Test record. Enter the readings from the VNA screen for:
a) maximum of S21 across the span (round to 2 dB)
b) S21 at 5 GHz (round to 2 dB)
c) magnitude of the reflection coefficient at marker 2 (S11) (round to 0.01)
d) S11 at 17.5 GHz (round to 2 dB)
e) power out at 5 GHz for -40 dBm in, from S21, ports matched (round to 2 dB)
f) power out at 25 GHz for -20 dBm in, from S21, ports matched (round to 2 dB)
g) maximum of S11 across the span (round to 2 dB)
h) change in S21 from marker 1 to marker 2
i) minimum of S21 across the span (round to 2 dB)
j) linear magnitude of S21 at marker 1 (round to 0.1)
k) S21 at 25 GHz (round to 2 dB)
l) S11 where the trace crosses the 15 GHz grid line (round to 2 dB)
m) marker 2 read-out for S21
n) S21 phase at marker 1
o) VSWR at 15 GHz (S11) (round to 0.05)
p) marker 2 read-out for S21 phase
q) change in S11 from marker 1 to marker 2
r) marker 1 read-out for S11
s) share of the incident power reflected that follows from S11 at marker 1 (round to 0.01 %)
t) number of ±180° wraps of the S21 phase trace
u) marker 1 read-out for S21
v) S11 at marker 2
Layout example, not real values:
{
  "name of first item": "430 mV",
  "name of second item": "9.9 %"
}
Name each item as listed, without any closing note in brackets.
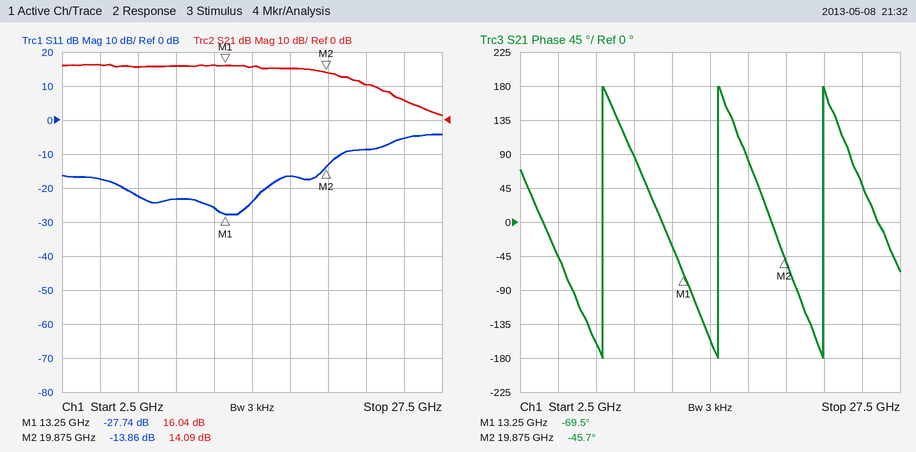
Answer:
{
  "maximum of S21 across the span": "16 dB",
  "S21 at 5 GHz": "16 dB",
  "magnitude of the reflection coefficient at marker 2 (S11)": "0.20",
  "S11 at 17.5 GHz": "-16 dB",
  "power out at 5 GHz for -40 dBm in, from S21, ports matched": "-24 dBm",
  "power out at 25 GHz for -20 dBm in, from S21, ports matched": "-14 dBm",
  "maximum of S11 across the span": "-4 dB",
  "change in S21 from marker 1 to marker 2": "-1.95 dB",
  "minimum of S21 across the span": "2 dB",
  "linear magnitude of S21 at marker 1": "6.3",
  "S21 at 25 GHz": "6 dB",
  "S11 where the trace crosses the 15 GHz grid line": "-24 dB",
  "marker 2 read-out for S21": "14.09 dB",
  "S21 phase at marker 1": "-69.5°",
  "VSWR at 15 GHz (S11)": "1.15",
  "marker 2 read-out for S21 phase": "-45.7°",
  "change in S11 from marker 1 to marker 2": "13.88 dB",
  "marker 1 read-out for S11": "-27.74 dB",
  "share of the incident power reflected that follows from S11 at marker 1": "0.17 %",
  "number of ±180° wraps of the S21 phase trace": "3",
  "marker 1 read-out for S21": "16.04 dB",
  "S11 at marker 2": "-13.86 dB"
}
